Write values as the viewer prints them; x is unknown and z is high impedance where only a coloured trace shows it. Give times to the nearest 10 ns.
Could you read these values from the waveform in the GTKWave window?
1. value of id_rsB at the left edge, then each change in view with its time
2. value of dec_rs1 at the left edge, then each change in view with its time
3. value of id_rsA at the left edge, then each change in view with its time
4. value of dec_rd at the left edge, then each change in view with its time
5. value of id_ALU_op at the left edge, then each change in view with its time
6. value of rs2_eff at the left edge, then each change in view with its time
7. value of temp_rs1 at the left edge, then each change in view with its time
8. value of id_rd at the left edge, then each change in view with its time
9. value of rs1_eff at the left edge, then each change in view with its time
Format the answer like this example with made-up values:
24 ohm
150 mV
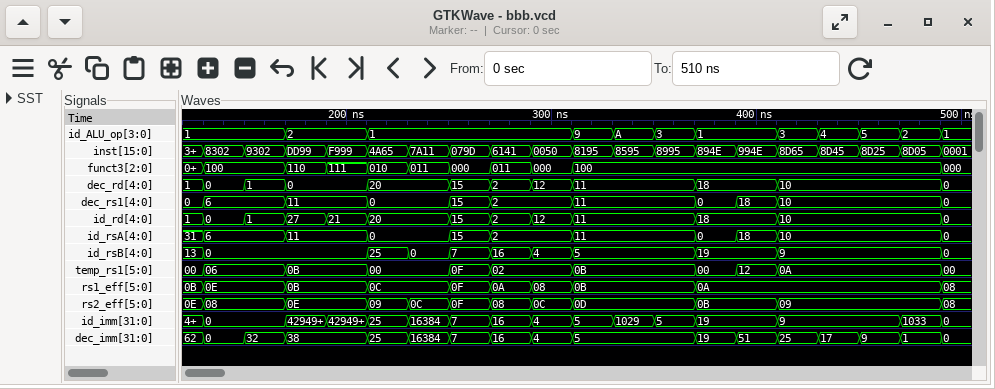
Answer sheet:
13, 0 at 130 ns, 25 at 210 ns, 0 at 230 ns, 7 at 250 ns, 16 at 270 ns, 4 at 290 ns, 5 at 310 ns, 19 at 370 ns, 9 at 410 ns, 0 at 490 ns
0, 6 at 130 ns, 11 at 170 ns, 0 at 210 ns, 15 at 250 ns, 2 at 270 ns, 11 at 310 ns, 0 at 370 ns, 18 at 390 ns, 10 at 410 ns, 0 at 490 ns
31, 6 at 130 ns, 11 at 170 ns, 0 at 210 ns, 15 at 250 ns, 2 at 270 ns, 11 at 310 ns, 0 at 370 ns, 18 at 390 ns, 10 at 410 ns, 0 at 490 ns
1, 0 at 130 ns, 1 at 150 ns, 0 at 170 ns, 20 at 210 ns, 15 at 250 ns, 2 at 270 ns, 12 at 290 ns, 11 at 310 ns, 18 at 370 ns, 10 at 410 ns, 0 at 490 ns
1, 2 at 170 ns, 1 at 210 ns, 9 at 310 ns, A at 330 ns, 3 at 350 ns, 1 at 370 ns, 3 at 410 ns, 4 at 430 ns, 5 at 450 ns, 2 at 470 ns, 1 at 490 ns
0E, 08 at 130 ns, 0E at 170 ns, 09 at 210 ns, 0C at 230 ns, 0F at 250 ns, 08 at 270 ns, 0C at 290 ns, 0D at 310 ns, 0B at 370 ns, 09 at 410 ns, 08 at 490 ns
00, 06 at 130 ns, 0B at 170 ns, 00 at 210 ns, 0F at 250 ns, 02 at 270 ns, 0B at 310 ns, 00 at 370 ns, 12 at 390 ns, 0A at 410 ns, 00 at 490 ns
1, 0 at 130 ns, 1 at 150 ns, 27 at 170 ns, 21 at 190 ns, 20 at 210 ns, 15 at 250 ns, 2 at 270 ns, 12 at 290 ns, 11 at 310 ns, 18 at 370 ns, 10 at 410 ns, 0 at 490 ns
0B, 0E at 130 ns, 0B at 170 ns, 0C at 210 ns, 0F at 250 ns, 0A at 270 ns, 08 at 290 ns, 0B at 310 ns, 0A at 370 ns, 08 at 490 ns
